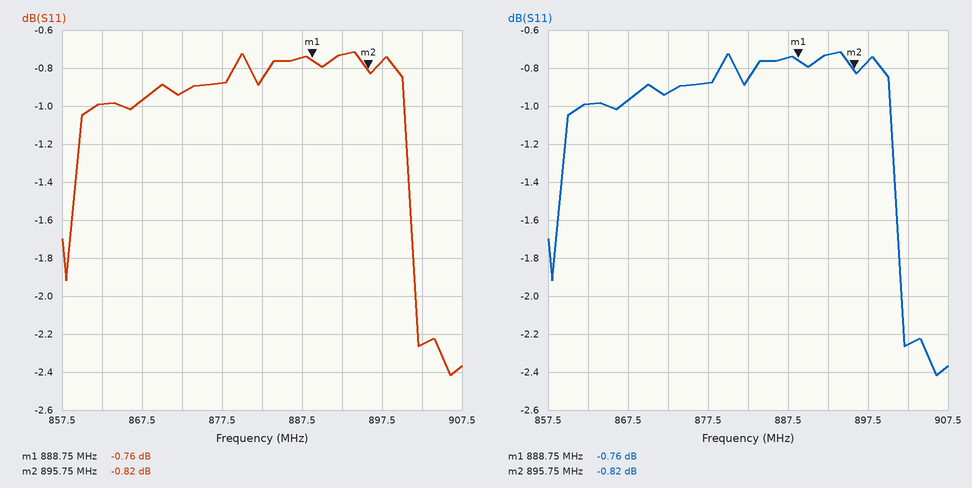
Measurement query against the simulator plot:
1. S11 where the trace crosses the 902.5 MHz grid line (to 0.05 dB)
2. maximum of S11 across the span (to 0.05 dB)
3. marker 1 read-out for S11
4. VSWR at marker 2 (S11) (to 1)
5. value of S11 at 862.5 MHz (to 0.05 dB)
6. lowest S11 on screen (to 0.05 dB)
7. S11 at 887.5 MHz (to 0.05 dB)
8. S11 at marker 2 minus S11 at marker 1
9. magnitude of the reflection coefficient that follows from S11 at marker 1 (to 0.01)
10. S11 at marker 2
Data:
-2.25 dB
-0.70 dB
-0.76 dB
21
-1.00 dB
-2.40 dB
-0.75 dB
-0.06 dB
0.92
-0.82 dB
